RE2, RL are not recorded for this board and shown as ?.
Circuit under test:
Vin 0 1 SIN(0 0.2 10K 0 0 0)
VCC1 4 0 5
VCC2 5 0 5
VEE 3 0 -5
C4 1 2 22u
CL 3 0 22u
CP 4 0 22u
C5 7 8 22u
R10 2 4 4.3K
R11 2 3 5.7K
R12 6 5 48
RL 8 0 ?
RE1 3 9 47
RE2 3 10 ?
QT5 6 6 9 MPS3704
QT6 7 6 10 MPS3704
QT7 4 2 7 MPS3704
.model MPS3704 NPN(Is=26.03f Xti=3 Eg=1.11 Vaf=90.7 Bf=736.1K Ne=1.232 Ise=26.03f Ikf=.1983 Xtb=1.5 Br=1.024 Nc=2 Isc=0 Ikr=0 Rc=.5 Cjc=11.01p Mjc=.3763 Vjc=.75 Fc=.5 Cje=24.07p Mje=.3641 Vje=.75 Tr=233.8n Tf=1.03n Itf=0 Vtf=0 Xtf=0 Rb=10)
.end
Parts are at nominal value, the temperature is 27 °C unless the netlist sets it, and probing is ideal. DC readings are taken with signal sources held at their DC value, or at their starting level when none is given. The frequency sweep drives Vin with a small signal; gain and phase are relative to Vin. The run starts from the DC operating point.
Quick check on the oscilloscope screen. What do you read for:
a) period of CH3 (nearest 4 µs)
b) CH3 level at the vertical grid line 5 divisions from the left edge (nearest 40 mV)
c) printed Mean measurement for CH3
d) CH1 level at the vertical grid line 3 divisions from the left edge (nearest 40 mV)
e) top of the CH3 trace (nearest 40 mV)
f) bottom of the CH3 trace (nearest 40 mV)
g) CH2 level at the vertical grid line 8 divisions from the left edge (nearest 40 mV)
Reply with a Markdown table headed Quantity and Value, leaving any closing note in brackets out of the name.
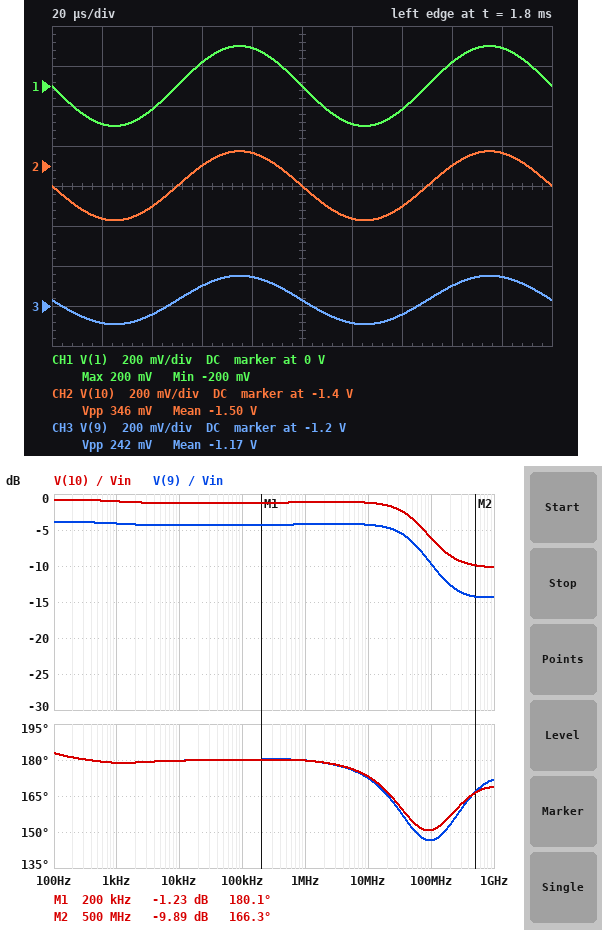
| Quantity | Value |
|---|---|
| period of CH3 | 100 µs |
| CH3 level at the vertical grid line 5 divisions from the left edge | -1.16 V |
| printed Mean measurement for CH3 | -1.17 V |
| CH1 level at the vertical grid line 3 divisions from the left edge | 120 mV |
| top of the CH3 trace | -1.04 V |
| bottom of the CH3 trace | -1.28 V |
| CH2 level at the vertical grid line 8 divisions from the left edge | -1.40 V |
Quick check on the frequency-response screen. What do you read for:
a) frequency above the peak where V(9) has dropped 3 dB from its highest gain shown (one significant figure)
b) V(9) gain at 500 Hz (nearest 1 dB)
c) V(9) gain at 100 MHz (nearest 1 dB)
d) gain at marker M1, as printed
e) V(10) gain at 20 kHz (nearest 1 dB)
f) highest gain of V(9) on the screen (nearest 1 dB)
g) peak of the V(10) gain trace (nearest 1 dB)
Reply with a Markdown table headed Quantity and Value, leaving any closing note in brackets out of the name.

| Quantity | Value |
|---|---|
| frequency above the peak where V(9) has dropped 3 dB from its highest gain shown | 50 MHz |
| V(9) gain at 500 Hz | -4 dB |
| V(9) gain at 100 MHz | -10 dB |
| gain at marker M1, as printed | -1.23 dB |
| V(10) gain at 20 kHz | -1 dB |
| highest gain of V(9) on the screen | -4 dB |
| peak of the V(10) gain trace | -1 dB |
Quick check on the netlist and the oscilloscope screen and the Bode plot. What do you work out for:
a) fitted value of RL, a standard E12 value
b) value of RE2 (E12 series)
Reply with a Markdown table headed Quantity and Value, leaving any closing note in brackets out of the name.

| Quantity | Value |
|---|---|
| fitted value of RL, a standard E12 value | 6.8 Ω |
| value of RE2 | 27 Ω |
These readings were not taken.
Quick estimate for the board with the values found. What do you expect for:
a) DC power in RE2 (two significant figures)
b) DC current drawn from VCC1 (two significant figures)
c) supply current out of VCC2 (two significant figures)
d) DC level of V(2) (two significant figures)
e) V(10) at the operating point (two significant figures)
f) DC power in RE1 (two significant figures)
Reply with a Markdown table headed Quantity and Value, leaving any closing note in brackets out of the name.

| Quantity | Value |
|---|---|
| DC power in RE2 | 450 mW |
| DC current drawn from VCC1 | 99 mA |
| supply current out of VCC2 | 110 mA |
| DC level of V(2) | -630 mV |
| V(10) at the operating point | -1.5 V |
| DC power in RE1 | 310 mW |
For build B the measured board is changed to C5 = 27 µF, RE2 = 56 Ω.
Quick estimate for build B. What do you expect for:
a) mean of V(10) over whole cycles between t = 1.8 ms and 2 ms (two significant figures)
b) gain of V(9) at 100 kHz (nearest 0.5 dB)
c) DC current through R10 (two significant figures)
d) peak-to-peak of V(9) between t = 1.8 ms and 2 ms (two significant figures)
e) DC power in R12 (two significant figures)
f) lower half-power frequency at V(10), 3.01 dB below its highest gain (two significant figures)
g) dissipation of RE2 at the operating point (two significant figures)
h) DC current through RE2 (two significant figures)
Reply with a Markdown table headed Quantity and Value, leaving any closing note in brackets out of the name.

| Quantity | Value |
|---|---|
| mean of V(10) over whole cycles between t = 1.8 ms and 2 ms | -910 mV |
| gain of V(9) at 100 kHz | -4.5 dB |
| DC current through R10 | 1.2 mA |
| peak-to-peak of V(9) between t = 1.8 ms and 2 ms | 230 mV |
| DC power in R12 | 520 mW |
| lower half-power frequency at V(10), 3.01 dB below its highest gain | 4.6 Hz |
| dissipation of RE2 at the operating point | 300 mW |
| DC current through RE2 | 73 mA |
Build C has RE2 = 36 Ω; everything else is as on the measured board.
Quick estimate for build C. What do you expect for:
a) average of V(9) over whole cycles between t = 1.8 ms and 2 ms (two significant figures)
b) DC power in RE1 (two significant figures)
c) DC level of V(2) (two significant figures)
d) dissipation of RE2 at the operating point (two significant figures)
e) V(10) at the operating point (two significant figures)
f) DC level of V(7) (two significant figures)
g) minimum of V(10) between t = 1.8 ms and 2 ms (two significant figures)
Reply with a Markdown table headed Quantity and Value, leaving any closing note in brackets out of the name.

| Quantity | Value |
|---|---|
| average of V(9) over whole cycles between t = 1.8 ms and 2 ms | -990 mV |
| DC power in RE1 | 340 mW |
| DC level of V(2) | -390 mV |
| dissipation of RE2 at the operating point | 390 mW |
| V(10) at the operating point | -1.2 V |
| DC level of V(7) | -1.1 V |
| minimum of V(10) between t = 1.8 ms and 2 ms | -1.4 V |
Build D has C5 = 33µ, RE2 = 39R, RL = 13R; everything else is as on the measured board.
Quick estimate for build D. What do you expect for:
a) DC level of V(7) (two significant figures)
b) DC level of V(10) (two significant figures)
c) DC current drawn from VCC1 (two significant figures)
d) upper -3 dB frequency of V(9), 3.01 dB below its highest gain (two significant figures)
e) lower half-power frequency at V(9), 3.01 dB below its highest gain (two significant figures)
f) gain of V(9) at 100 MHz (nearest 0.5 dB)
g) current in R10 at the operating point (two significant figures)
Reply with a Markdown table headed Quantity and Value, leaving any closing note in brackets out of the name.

| Quantity | Value |
|---|---|
| DC level of V(7) | -1.1 V |
| DC level of V(10) | -1.2 V |
| DC current drawn from VCC1 | 77 mA |
| upper -3 dB frequency of V(9), 3.01 dB below its highest gain | 81 MHz |
| lower half-power frequency at V(9), 3.01 dB below its highest gain | 5.0 Hz |
| gain of V(9) at 100 MHz | -7.5 dB |
| current in R10 at the operating point | 1.2 mA |
